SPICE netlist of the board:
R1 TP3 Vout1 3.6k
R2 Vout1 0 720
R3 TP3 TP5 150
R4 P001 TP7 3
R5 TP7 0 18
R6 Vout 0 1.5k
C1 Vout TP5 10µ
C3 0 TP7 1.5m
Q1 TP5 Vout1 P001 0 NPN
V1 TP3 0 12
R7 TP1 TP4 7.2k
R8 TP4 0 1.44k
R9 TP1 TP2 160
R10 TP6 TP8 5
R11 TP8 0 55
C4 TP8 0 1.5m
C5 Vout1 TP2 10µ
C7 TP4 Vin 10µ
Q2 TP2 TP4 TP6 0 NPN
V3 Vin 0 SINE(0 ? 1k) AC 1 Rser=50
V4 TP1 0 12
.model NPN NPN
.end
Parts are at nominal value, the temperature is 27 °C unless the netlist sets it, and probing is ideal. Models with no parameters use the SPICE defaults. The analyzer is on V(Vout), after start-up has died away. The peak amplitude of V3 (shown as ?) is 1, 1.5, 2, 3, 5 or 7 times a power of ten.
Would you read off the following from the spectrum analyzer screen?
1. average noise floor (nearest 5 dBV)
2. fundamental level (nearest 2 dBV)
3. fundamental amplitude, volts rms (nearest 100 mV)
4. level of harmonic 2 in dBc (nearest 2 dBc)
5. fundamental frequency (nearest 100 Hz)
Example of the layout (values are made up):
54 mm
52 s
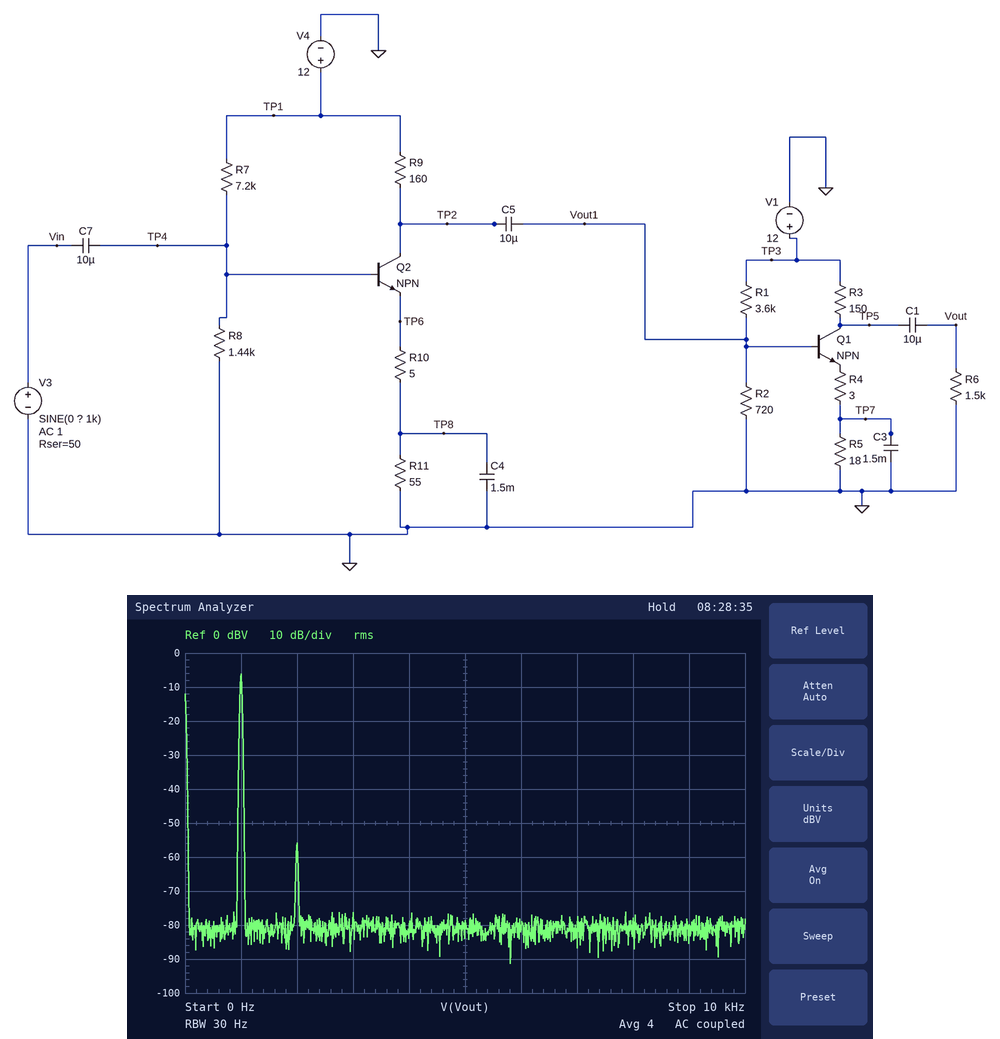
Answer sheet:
-80 dBV
-6 dBV
500 mV
-50 dBc
1.0 kHz
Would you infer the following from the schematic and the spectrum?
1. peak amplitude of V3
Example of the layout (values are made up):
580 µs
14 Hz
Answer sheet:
1.5 mV
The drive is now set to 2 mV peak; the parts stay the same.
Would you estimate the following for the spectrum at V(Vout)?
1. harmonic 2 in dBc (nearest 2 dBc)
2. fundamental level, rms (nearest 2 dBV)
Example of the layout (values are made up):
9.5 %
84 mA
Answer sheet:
-48 dBc
-4 dBV
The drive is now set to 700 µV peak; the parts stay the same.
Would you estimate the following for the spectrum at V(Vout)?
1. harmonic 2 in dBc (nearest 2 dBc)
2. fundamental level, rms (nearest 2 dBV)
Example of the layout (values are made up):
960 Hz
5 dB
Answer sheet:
-56 dBc
-12 dBV
